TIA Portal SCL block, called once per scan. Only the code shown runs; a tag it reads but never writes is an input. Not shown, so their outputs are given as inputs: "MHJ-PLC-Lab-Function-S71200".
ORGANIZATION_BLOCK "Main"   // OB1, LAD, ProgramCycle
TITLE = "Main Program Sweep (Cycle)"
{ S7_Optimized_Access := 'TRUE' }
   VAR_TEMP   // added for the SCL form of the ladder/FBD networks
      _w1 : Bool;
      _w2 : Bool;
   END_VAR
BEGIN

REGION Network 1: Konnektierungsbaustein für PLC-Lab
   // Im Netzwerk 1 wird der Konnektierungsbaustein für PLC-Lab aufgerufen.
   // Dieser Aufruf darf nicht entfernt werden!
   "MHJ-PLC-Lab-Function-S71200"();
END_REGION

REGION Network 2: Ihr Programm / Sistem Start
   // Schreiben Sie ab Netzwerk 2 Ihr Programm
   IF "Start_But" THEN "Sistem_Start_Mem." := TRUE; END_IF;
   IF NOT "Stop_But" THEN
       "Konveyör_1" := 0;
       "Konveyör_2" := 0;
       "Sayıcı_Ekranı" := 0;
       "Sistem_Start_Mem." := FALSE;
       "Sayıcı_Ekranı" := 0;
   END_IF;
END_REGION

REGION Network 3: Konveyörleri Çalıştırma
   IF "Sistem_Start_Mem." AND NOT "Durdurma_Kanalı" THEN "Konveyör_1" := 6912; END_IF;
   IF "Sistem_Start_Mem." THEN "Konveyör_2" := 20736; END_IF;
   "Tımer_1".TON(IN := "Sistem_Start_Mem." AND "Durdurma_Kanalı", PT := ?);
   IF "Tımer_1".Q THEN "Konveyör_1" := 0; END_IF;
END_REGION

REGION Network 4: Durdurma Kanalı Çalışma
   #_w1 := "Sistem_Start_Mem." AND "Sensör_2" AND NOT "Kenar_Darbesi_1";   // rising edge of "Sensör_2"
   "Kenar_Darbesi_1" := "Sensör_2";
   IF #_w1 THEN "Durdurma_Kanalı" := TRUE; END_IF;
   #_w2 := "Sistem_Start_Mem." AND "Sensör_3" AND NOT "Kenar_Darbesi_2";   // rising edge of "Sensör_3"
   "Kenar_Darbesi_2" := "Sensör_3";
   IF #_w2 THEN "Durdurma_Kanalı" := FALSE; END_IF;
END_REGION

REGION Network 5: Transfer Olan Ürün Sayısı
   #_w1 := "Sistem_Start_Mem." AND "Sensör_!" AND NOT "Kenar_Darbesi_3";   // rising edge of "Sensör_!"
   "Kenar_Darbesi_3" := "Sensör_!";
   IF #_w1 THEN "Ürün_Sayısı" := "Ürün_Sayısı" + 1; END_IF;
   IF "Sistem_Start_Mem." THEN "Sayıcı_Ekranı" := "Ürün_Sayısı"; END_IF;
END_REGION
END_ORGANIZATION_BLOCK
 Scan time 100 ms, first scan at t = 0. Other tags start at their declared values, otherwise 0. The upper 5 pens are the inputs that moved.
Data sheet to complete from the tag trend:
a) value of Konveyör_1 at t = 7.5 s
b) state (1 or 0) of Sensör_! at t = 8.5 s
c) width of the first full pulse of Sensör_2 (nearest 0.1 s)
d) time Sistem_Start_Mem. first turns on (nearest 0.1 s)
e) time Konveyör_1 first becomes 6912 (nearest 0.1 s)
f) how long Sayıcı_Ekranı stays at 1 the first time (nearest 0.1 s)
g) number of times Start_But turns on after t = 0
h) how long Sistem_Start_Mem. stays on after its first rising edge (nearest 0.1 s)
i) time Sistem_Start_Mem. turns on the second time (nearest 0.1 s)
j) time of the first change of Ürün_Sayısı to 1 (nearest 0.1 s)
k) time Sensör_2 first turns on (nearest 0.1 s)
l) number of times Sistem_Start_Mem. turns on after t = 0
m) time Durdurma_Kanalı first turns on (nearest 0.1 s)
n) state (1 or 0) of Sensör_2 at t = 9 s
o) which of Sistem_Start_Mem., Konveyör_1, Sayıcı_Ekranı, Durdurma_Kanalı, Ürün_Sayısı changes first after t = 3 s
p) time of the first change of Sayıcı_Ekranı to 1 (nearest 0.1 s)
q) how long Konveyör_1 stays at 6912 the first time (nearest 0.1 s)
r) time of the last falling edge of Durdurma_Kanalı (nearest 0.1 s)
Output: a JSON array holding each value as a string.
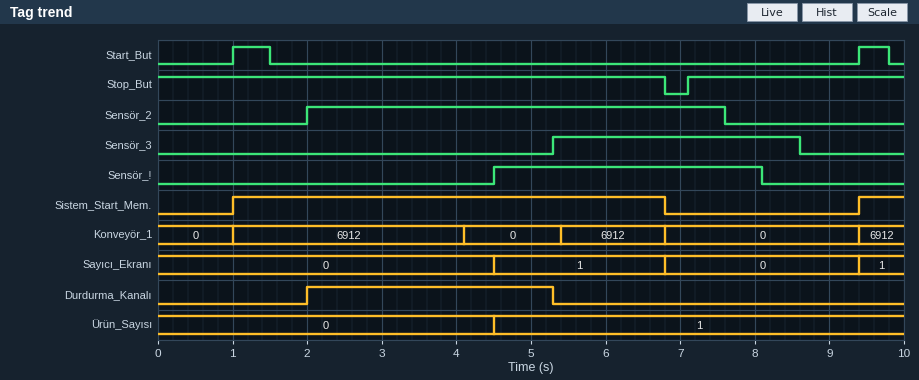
["0", "0", "5.6 s", "1.0 s", "1.0 s", "2.3 s", "2", "5.8 s", "9.4 s", "4.5 s", "2.0 s", "2", "2.0 s", "0", "Konveyör_1", "4.5 s", "3.1 s", "5.3 s"]
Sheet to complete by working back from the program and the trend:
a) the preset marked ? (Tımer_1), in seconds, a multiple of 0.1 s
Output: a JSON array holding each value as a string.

["2.0 s"]
